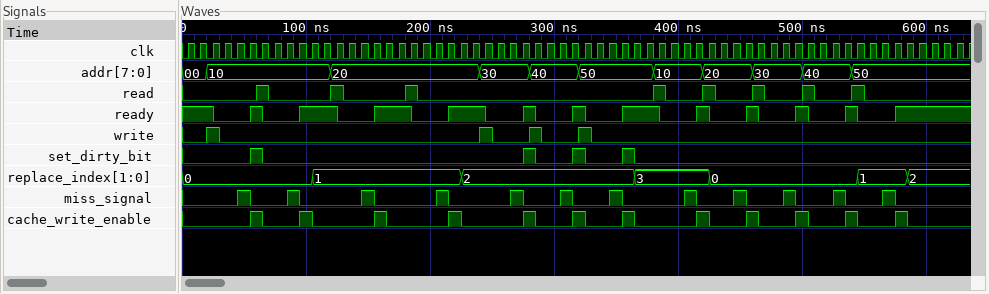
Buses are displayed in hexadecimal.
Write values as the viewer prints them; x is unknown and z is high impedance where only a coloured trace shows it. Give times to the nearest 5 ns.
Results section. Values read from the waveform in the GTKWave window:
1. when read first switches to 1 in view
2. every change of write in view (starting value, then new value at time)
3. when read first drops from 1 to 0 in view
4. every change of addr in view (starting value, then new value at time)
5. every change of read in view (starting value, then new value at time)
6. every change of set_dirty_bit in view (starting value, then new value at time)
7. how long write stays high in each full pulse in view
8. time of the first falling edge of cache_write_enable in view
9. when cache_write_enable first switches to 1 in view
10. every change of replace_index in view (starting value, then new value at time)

60 ns
0, 1 at 20 ns, 0 at 30 ns, 1 at 240 ns, 0 at 250 ns, 1 at 280 ns, 0 at 290 ns, 1 at 320 ns, 0 at 330 ns
70 ns
00, 10 at 20 ns, 20 at 120 ns, 30 at 240 ns, 40 at 280 ns, 50 at 320 ns, 10 at 380 ns, 20 at 420 ns, 30 at 460 ns, 40 at 500 ns, 50 at 540 ns
0, 1 at 60 ns, 0 at 70 ns, 1 at 120 ns, 0 at 130 ns, 1 at 180 ns, 0 at 190 ns, 1 at 380 ns, 0 at 390 ns, 1 at 420 ns, 0 at 430 ns, 1 at 460 ns, 0 at 470 ns, 1 at 500 ns, 0 at 510 ns, 1 at 540 ns, 0 at 550 ns
0, 1 at 55 ns, 0 at 65 ns, 1 at 275 ns, 0 at 285 ns, 1 at 315 ns, 0 at 325 ns, 1 at 355 ns, 0 at 365 ns
10 ns, 10 ns, 10 ns, 10 ns
65 ns
55 ns
0, 1 at 105 ns, 2 at 225 ns, 3 at 365 ns, 0 at 425 ns, 1 at 545 ns, 2 at 585 ns
